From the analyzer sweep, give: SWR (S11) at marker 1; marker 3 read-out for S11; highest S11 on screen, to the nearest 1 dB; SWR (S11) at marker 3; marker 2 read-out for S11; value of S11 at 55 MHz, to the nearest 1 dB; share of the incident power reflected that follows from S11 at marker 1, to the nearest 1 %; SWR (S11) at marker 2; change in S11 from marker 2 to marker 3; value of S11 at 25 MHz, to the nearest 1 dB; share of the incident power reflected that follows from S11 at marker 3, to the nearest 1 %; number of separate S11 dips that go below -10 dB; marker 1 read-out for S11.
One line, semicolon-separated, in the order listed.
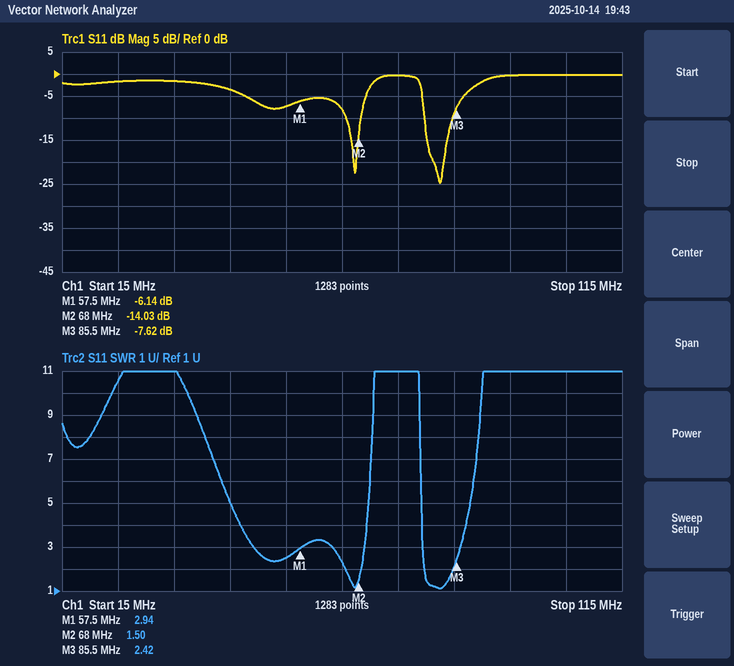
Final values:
2.94; -7.62 dB; 0 dB; 2.42; -14.03 dB; -7 dB; 24 %; 1.50; 6.41 dB; -2 dB; 17 %; 2; -6.14 dB
